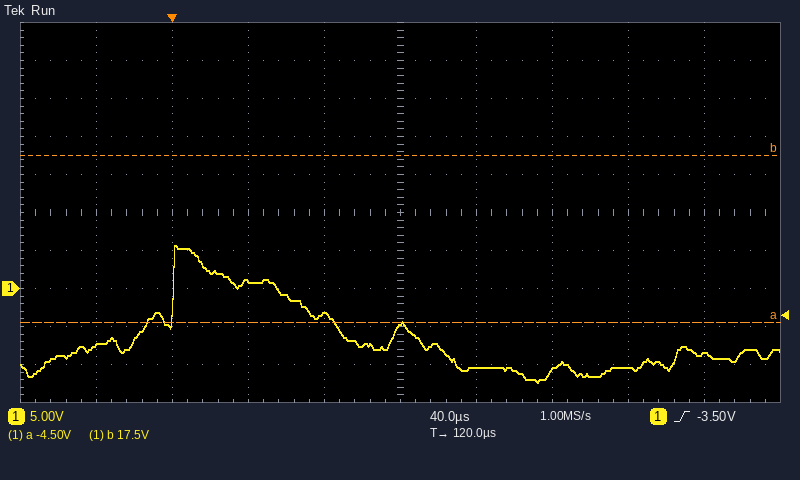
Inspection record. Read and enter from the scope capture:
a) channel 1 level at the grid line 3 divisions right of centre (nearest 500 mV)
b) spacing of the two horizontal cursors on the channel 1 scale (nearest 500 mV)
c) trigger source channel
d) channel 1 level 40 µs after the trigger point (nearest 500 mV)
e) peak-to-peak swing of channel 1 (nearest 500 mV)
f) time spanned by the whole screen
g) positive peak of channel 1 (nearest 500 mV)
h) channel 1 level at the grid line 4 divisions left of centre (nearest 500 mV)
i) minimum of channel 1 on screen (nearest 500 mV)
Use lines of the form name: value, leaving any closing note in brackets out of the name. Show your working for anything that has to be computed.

channel 1 level at the grid line 3 divisions right of centre: -10.5 V
spacing of the two horizontal cursors on the channel 1 scale: 22.0 V
trigger source channel: channel 1
channel 1 level 40 µs after the trigger point: 1.0 V
peak-to-peak swing of channel 1: 5.5 V − (-12.5 V) = 18.0 V
time spanned by the whole screen: 400 µs
positive peak of channel 1: 5.5 V
channel 1 level at the grid line 4 divisions left of centre: -7.5 V
minimum of channel 1 on screen: -12.5 V
